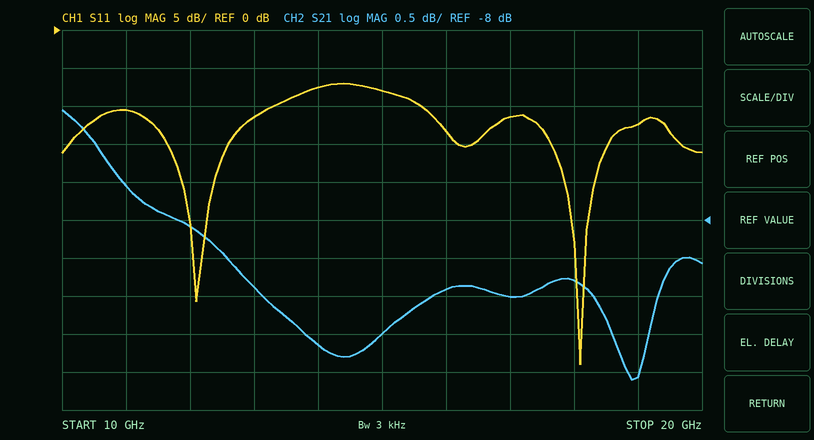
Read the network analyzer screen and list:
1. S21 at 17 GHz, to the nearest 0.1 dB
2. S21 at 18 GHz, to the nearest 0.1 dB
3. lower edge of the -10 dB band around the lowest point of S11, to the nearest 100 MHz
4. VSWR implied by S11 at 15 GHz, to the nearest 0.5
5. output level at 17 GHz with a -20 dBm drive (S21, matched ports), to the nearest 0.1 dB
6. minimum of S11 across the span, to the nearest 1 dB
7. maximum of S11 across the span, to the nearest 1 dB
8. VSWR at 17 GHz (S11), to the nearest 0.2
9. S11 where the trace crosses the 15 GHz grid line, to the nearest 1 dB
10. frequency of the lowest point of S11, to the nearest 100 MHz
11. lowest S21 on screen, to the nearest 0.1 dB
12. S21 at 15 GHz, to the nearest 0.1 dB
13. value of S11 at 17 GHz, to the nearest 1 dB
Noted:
-9.0 dB
-8.8 dB
15.6 GHz
2.5
-29.0 dBm
-44 dB
-7 dB
1.8
-8 dB
18.1 GHz
-10.1 dB
-9.5 dB
-11 dB
